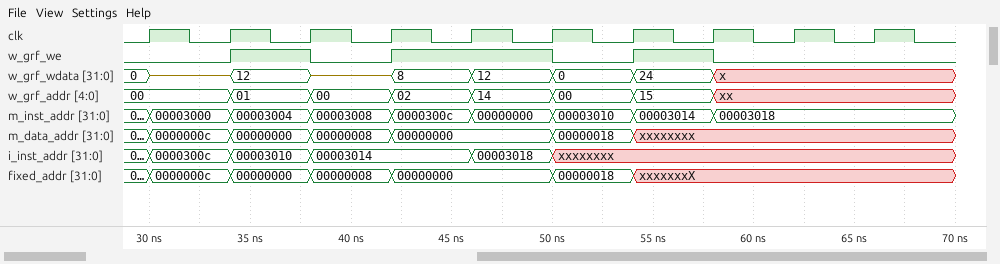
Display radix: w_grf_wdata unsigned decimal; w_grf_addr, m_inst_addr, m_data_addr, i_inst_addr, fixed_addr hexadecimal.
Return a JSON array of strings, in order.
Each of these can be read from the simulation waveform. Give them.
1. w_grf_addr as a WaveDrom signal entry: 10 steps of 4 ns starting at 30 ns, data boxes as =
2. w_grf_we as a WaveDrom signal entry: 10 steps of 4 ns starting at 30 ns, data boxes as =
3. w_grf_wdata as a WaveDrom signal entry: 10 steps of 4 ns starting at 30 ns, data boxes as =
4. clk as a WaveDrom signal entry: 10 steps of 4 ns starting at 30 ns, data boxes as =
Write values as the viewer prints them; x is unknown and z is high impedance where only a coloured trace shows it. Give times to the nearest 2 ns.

["{name: 'w_grf_addr', wave: '=======x..', data: '00 01 00 02 14 00 15'}", "{name: 'w_grf_we', wave: '0101.010..'}", "{name: 'w_grf_wdata', wave: 'z=z====x..', data: '12 8 12 0 24'}", "{name: 'clk', wave: 'p.........'}"]
